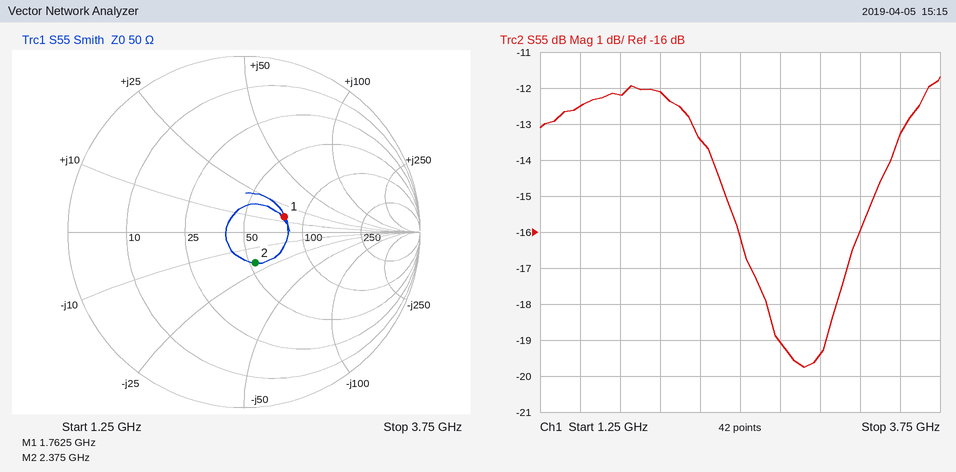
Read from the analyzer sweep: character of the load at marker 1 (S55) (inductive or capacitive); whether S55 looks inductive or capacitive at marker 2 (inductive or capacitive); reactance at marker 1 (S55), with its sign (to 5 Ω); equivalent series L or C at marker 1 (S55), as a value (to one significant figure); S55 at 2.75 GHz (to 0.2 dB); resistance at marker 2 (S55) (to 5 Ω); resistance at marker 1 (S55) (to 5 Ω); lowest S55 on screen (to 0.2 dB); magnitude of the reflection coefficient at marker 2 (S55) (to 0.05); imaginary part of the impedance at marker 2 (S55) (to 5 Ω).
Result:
inductive
capacitive
+15 Ω
1 nH
-19.0 dB
55 Ω
80 Ω
-19.8 dB
0.20
-20 Ω
